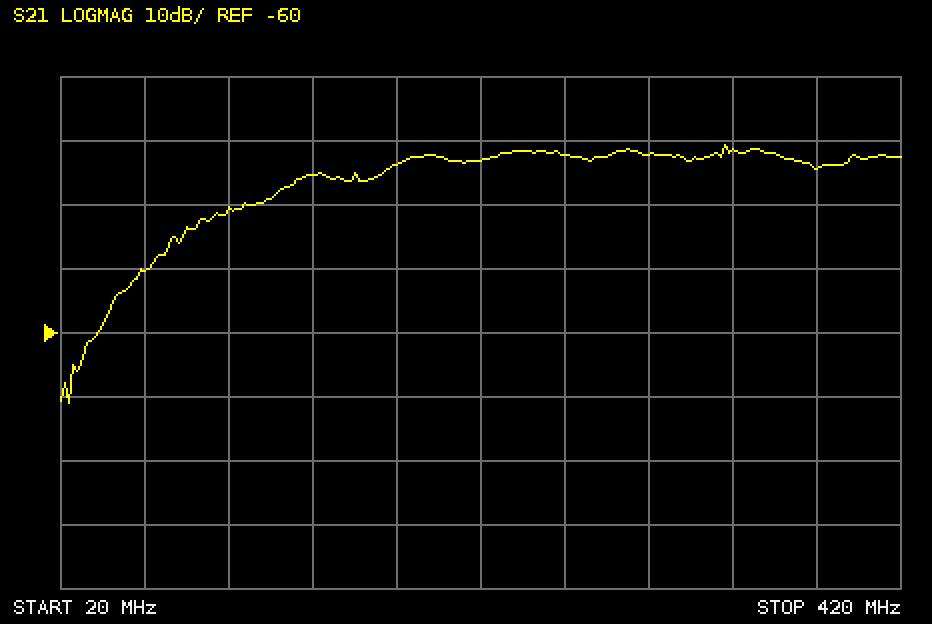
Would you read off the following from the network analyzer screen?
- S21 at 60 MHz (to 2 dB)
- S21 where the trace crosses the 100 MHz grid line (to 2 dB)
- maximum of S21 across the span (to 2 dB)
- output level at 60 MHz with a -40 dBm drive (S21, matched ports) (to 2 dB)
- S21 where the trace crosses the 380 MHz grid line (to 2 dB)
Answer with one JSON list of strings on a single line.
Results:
["-50 dB", "-40 dB", "-30 dB", "-90 dBm", "-34 dB"]
